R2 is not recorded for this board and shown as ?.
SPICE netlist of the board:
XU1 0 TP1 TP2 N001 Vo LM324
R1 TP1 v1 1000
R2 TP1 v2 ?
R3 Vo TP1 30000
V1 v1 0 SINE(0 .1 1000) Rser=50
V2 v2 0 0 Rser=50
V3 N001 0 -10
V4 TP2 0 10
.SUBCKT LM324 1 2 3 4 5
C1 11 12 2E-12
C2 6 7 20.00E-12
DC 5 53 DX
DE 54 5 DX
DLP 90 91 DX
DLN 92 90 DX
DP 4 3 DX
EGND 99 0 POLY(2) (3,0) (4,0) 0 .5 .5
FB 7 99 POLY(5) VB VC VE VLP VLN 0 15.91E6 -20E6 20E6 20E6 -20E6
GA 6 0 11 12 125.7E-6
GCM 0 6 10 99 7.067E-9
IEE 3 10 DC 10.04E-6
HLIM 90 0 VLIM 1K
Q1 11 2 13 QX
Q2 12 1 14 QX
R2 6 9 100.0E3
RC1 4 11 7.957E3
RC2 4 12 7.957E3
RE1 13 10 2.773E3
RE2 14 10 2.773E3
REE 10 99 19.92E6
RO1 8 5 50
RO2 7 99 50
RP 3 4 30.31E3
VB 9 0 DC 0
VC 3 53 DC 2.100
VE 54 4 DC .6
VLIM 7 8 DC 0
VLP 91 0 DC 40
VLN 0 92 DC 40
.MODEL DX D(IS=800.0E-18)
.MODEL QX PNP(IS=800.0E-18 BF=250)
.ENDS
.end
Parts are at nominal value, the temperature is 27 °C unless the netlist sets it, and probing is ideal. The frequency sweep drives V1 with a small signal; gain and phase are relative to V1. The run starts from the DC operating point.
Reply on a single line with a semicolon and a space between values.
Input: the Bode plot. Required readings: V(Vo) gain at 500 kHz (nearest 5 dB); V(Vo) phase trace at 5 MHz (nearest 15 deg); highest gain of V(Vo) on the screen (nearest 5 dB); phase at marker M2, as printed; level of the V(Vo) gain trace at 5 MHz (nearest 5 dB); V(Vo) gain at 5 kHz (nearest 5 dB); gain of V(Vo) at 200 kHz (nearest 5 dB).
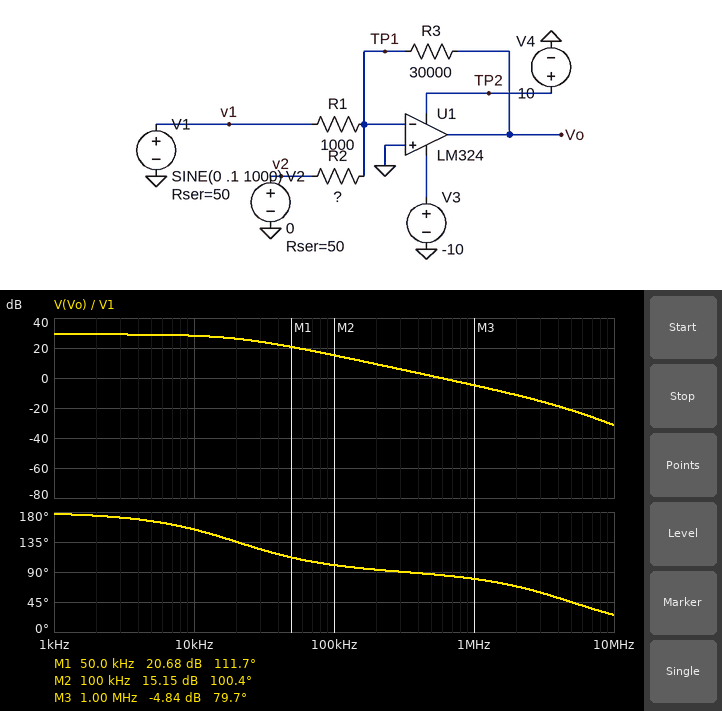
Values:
0 dB; 45 deg; 30 dB; 100.4 deg; -20 dB; 30 dB; 10 dB
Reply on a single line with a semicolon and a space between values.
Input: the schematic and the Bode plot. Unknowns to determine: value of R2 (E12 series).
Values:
1.5 kΩ
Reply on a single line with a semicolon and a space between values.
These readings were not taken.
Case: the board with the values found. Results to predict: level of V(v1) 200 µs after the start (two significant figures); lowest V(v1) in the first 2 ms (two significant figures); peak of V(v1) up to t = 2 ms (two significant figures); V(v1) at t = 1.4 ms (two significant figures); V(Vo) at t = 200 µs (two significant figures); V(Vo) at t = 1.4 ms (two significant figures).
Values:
91 mV; -95 mV; 95 mV; 56 mV; -2.7 V; -1.8 V
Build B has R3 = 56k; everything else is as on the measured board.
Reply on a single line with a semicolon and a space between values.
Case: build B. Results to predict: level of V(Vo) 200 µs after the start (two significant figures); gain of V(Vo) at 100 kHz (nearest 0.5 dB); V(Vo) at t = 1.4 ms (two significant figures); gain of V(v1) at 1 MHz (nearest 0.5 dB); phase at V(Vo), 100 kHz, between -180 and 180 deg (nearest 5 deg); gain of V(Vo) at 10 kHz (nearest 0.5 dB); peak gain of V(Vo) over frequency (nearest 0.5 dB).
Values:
-4.9 V; 15.5 dB; -3.5 V; 0 dB; 95 deg; 32.0 dB; 34.5 dB
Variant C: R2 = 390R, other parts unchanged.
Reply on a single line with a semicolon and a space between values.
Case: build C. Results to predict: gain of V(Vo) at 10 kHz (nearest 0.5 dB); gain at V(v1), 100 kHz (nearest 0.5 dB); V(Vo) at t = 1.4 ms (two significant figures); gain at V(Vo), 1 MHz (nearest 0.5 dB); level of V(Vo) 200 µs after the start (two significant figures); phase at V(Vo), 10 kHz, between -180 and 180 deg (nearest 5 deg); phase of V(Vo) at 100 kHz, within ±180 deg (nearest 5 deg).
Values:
26.0 dB; -0.5 dB; -1.9 V; -11.0 dB; -2.6 V; 135 deg; 95 deg
